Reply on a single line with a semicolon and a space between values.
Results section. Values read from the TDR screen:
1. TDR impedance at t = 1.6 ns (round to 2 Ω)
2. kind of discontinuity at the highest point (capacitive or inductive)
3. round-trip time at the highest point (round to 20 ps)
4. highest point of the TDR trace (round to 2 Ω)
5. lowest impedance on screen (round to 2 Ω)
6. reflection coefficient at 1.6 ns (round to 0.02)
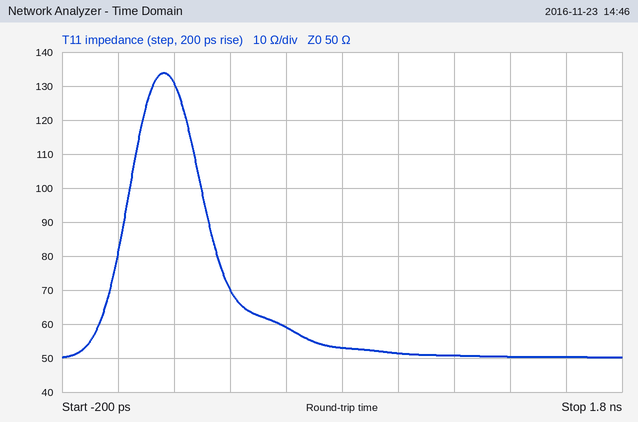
50 Ω; inductive; 160 ps; 134 Ω; 50 Ω; 0.00
